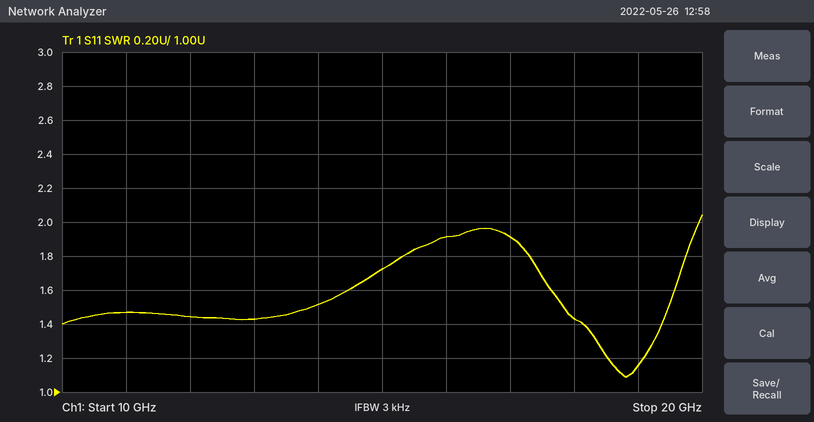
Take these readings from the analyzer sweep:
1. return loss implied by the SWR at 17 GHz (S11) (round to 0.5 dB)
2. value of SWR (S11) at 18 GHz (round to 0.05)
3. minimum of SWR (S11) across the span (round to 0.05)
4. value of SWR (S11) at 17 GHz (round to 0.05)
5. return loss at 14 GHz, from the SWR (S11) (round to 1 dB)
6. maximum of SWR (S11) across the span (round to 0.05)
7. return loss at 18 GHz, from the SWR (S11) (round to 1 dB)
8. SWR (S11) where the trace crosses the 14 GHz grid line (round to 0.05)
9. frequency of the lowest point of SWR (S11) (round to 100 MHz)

10.0 dB
1.45
1.10
1.90
14 dB
2.05
15 dB
1.50
18.8 GHz
